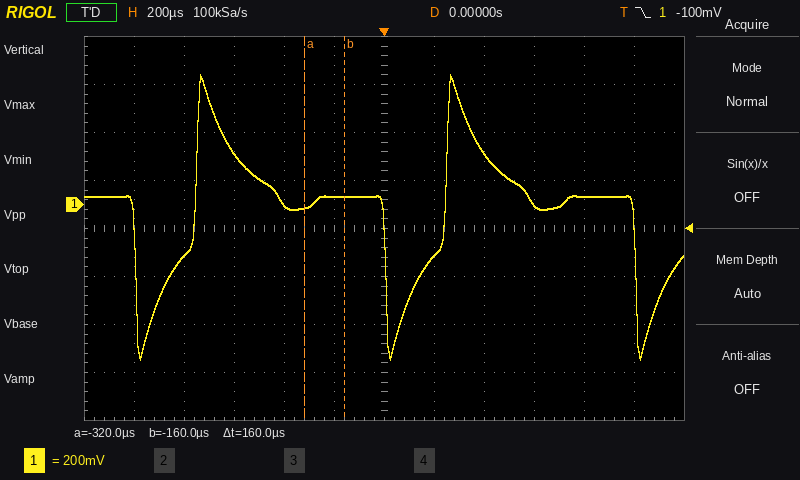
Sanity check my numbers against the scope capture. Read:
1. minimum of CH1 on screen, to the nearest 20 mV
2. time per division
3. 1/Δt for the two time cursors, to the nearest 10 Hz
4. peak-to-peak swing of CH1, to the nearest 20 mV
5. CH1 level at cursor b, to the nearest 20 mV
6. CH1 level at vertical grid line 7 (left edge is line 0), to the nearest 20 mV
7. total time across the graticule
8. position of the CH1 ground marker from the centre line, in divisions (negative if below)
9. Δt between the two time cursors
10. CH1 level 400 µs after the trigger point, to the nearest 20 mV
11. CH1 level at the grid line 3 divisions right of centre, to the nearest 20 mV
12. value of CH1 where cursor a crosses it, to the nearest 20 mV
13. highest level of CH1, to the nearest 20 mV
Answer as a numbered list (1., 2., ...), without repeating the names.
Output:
1. -640 mV
2. 200 µs
3. 6.25 kHz
4. 1.18 V
5. 40 mV
6. -220 mV
7. 2.4 ms
8. +0.5 div
9. 160 µs
10. 220 mV
11. 0 mV
12. -20 mV
13. 540 mV
